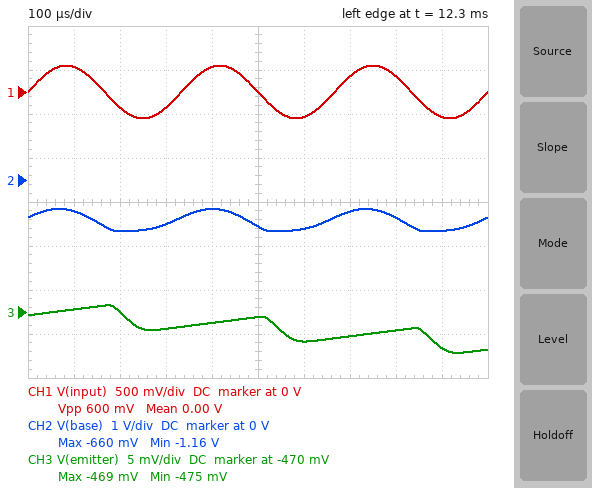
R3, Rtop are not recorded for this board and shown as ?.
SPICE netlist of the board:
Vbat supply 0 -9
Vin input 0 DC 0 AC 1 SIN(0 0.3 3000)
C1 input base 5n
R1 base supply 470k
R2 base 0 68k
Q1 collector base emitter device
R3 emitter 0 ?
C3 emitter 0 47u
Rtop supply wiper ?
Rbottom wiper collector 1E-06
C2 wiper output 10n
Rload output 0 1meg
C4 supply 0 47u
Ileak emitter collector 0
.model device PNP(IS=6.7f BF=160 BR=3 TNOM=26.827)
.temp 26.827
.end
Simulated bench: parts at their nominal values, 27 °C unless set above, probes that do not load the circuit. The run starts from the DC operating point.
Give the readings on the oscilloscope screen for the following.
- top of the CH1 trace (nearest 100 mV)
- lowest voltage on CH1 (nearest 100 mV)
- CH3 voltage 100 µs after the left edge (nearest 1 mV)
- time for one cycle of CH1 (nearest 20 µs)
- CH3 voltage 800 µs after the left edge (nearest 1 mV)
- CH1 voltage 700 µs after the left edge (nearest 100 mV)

300 mV
-300 mV
-470 mV
340 µs
-472 mV
200 mV
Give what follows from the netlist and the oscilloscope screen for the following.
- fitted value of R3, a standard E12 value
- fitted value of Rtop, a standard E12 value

1.5 kΩ
3.3 kΩ
